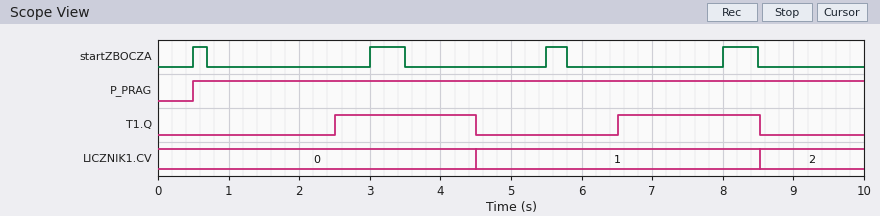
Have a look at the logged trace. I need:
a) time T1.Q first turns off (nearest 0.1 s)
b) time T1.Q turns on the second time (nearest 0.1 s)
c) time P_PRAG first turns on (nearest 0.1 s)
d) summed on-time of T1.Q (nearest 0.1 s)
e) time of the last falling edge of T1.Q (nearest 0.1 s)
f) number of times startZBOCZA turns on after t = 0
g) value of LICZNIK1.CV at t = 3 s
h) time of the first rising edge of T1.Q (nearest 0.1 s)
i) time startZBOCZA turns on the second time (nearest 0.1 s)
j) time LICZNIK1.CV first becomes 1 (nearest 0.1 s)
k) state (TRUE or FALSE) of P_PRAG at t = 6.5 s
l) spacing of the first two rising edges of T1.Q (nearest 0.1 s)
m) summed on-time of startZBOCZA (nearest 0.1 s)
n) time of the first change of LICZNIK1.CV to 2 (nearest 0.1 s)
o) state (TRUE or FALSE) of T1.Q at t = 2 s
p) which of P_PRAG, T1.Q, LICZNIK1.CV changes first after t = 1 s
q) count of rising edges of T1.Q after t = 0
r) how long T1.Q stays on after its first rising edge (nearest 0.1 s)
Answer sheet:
4.5 s
6.5 s
0.5 s
4.0 s
8.5 s
4
0
2.5 s
3.0 s
4.5 s
TRUE
4.0 s
1.5 s
8.5 s
FALSE
T1.Q
2
2.0 s
